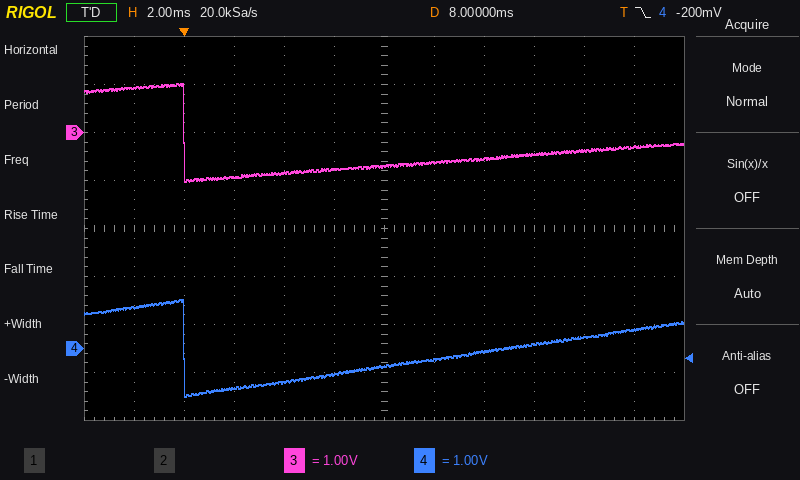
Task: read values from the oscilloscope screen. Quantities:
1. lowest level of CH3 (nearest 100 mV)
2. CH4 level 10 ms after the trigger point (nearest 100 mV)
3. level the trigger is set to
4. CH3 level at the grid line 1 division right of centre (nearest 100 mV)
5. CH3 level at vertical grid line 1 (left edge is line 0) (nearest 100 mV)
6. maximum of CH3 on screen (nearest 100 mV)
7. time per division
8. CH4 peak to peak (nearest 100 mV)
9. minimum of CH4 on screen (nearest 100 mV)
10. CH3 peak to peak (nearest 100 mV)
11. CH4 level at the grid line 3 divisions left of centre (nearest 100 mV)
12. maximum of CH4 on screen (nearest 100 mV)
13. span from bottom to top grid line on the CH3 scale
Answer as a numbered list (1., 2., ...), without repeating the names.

1. -1.0 V
2. -200 mV
3. -200 mV
4. -600 mV
5. 900 mV
6. 1.0 V
7. 2 ms
8. 2.0 V
9. -1.0 V
10. 2.0 V
11. -800 mV
12. 1.0 V
13. 8 V
